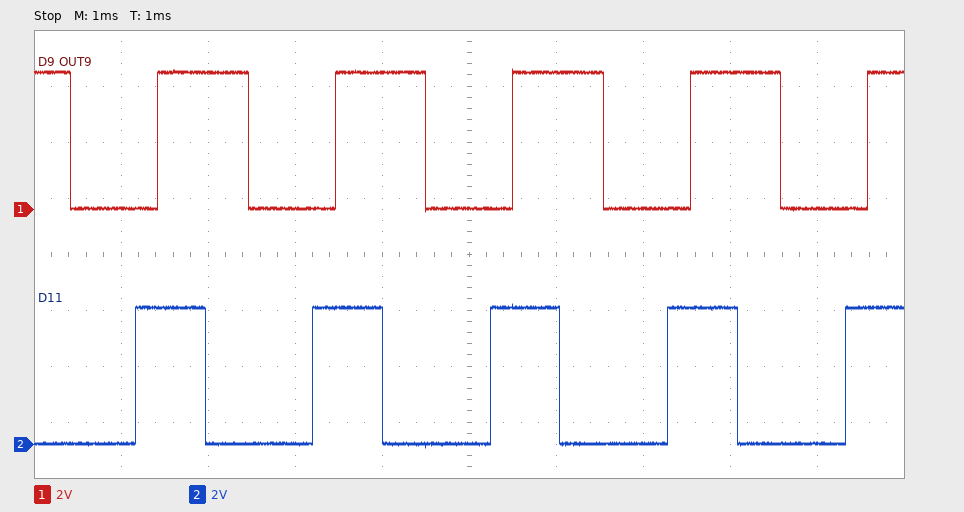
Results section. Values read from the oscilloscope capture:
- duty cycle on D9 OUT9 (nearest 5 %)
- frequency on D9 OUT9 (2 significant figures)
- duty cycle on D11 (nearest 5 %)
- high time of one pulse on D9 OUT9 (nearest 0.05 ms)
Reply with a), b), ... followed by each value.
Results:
a) 50 %
b) 490 Hz
c) 40 %
d) 1.05 ms
